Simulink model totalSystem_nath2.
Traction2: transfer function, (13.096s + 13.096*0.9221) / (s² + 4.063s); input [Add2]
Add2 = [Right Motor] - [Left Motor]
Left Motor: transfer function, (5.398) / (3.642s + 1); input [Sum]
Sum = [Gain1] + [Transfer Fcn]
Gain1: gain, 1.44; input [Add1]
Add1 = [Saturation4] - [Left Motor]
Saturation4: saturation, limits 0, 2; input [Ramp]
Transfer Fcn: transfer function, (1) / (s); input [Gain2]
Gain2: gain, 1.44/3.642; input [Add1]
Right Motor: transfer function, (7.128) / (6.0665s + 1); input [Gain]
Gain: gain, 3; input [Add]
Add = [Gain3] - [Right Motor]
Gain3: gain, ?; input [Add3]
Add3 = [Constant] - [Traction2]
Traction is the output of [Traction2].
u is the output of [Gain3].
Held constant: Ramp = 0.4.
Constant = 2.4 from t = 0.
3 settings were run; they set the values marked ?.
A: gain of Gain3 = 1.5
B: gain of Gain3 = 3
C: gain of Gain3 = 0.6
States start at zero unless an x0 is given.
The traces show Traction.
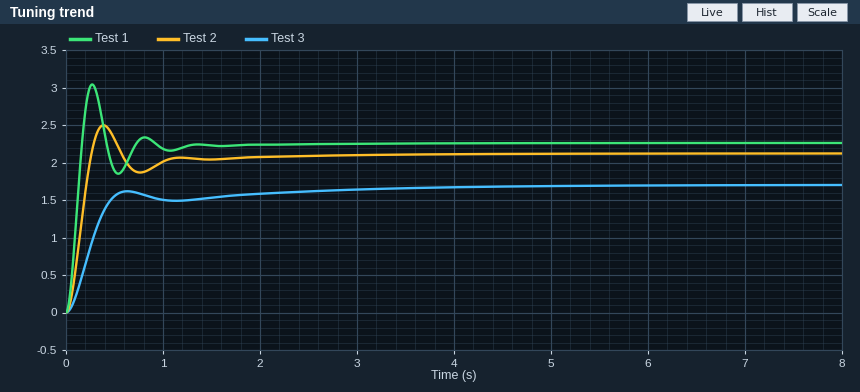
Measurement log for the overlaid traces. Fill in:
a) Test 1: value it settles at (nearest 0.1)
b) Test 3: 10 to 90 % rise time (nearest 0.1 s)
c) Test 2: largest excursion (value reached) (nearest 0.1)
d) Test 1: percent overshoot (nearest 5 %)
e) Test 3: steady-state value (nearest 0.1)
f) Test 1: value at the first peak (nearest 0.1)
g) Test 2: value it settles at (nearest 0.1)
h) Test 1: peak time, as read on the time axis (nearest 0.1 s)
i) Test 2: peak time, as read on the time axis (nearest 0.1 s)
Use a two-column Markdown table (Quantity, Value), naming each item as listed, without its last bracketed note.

| Quantity | Value |
|---|---|
| Test 1: value it settles at | 2.3 |
| Test 3: 10 to 90 % rise time | 0.4 s |
| Test 2: largest excursion (value reached) | 2.5 |
| Test 1: percent overshoot | 35 % |
| Test 3: steady-state value | 1.7 |
| Test 1: value at the first peak | 3.0 |
| Test 2: value it settles at | 2.1 |
| Test 1: peak time, as read on the time axis | 0.3 s |
| Test 2: peak time, as read on the time axis | 0.4 s |
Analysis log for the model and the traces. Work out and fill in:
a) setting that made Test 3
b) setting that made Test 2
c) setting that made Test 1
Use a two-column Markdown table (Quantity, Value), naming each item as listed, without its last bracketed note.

| Quantity | Value |
|---|---|
| setting that made Test 3 | C |
| setting that made Test 2 | A |
| setting that made Test 1 | B |
